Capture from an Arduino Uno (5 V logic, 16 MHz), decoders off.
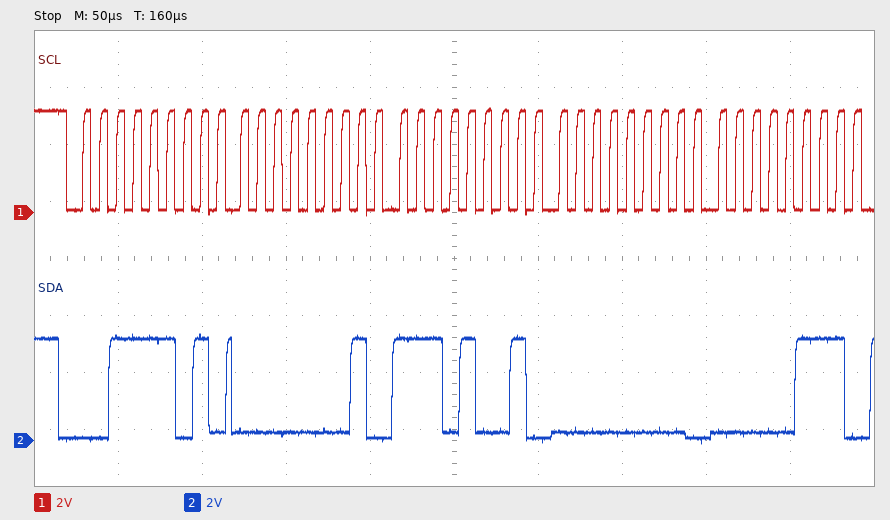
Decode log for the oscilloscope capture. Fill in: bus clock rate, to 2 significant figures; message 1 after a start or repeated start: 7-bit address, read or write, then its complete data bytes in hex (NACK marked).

100 kHz
0x1E read: 01 E9 00 07
